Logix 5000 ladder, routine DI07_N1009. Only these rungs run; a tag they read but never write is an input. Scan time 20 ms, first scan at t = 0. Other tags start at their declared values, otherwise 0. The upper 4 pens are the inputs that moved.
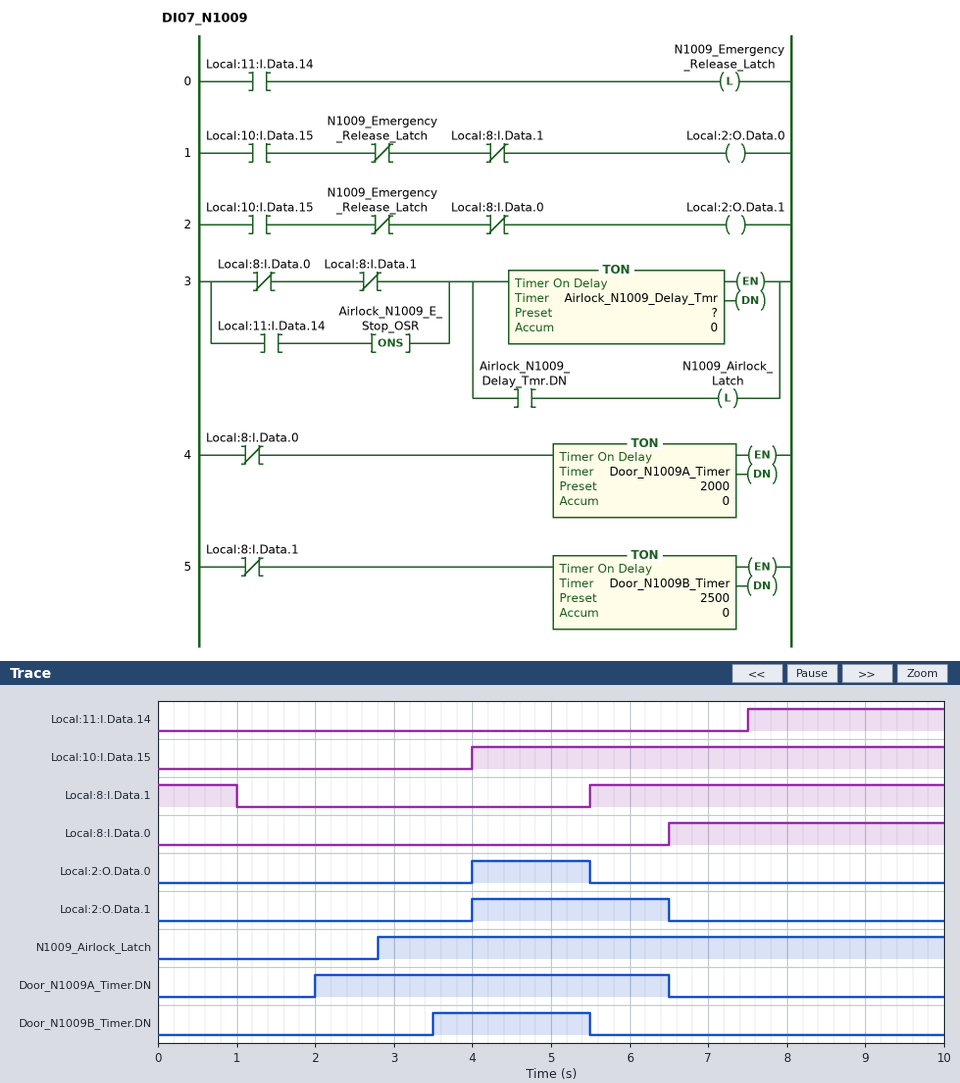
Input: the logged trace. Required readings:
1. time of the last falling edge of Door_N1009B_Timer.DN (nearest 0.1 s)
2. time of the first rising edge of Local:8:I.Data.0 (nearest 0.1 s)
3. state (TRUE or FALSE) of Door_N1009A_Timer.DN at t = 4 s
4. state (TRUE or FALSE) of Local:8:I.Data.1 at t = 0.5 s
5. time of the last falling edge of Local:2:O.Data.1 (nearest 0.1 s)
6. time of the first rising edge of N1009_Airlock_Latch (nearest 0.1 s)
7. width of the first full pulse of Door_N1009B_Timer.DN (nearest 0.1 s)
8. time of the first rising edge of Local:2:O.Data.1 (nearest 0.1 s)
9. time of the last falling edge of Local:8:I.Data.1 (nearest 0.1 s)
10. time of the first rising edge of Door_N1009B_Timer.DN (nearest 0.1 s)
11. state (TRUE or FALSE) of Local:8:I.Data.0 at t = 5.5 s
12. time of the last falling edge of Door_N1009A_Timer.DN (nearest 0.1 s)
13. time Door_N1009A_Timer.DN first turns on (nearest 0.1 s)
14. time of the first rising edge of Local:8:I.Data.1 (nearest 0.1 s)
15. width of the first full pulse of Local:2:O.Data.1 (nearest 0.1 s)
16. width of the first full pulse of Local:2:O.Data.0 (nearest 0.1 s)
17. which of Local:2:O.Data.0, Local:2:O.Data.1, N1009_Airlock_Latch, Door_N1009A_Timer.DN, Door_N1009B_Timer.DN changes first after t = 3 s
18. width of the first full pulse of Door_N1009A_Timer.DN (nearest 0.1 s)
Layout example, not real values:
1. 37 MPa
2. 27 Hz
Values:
1. 5.5 s
2. 6.5 s
3. TRUE
4. TRUE
5. 6.5 s
6. 2.8 s
7. 2.0 s
8. 4.0 s
9. 1.0 s
10. 3.5 s
11. FALSE
12. 6.5 s
13. 2.0 s
14. 5.5 s
15. 2.5 s
16. 1.5 s
17. Door_N1009B_Timer.DN
18. 4.5 s
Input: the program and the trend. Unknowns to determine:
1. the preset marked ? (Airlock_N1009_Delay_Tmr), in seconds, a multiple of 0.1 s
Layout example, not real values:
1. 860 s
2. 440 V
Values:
1. 1.8 s
